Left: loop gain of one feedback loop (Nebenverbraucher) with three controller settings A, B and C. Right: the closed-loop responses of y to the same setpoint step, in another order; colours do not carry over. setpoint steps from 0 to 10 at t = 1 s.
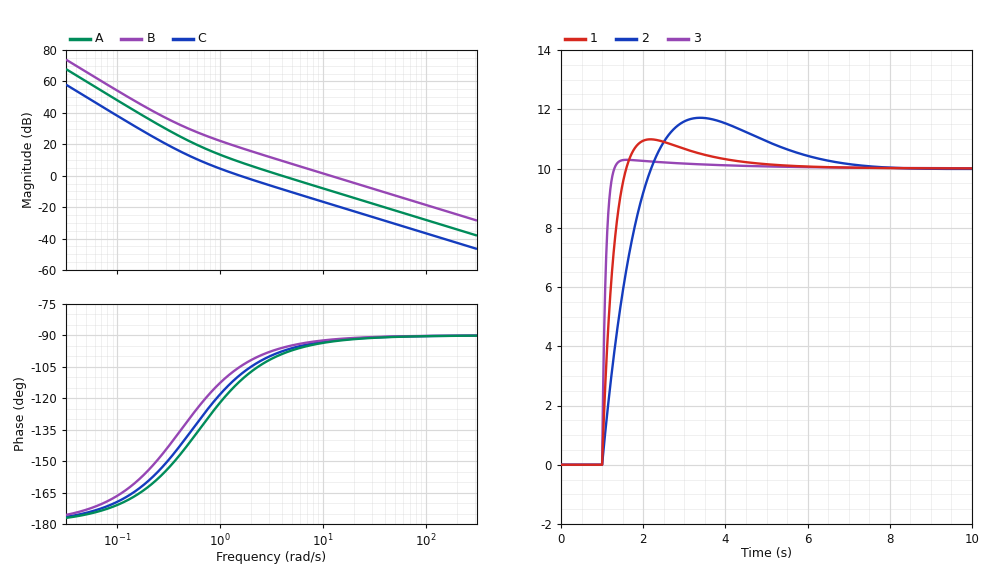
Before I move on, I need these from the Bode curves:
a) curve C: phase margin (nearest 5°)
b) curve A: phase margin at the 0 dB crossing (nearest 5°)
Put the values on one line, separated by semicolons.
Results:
70°; 80°
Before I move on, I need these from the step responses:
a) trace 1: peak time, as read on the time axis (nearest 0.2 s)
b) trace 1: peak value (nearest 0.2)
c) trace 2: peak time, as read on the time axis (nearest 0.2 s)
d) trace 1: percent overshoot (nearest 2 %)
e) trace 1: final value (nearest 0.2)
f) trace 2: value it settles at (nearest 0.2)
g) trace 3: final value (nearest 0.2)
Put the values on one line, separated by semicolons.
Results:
2.2 s; 11.0; 3.4 s; 10 %; 10.0; 10.0; 10.0
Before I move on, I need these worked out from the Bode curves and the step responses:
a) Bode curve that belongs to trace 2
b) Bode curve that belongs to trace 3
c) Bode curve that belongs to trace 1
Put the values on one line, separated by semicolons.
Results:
C; B; A
